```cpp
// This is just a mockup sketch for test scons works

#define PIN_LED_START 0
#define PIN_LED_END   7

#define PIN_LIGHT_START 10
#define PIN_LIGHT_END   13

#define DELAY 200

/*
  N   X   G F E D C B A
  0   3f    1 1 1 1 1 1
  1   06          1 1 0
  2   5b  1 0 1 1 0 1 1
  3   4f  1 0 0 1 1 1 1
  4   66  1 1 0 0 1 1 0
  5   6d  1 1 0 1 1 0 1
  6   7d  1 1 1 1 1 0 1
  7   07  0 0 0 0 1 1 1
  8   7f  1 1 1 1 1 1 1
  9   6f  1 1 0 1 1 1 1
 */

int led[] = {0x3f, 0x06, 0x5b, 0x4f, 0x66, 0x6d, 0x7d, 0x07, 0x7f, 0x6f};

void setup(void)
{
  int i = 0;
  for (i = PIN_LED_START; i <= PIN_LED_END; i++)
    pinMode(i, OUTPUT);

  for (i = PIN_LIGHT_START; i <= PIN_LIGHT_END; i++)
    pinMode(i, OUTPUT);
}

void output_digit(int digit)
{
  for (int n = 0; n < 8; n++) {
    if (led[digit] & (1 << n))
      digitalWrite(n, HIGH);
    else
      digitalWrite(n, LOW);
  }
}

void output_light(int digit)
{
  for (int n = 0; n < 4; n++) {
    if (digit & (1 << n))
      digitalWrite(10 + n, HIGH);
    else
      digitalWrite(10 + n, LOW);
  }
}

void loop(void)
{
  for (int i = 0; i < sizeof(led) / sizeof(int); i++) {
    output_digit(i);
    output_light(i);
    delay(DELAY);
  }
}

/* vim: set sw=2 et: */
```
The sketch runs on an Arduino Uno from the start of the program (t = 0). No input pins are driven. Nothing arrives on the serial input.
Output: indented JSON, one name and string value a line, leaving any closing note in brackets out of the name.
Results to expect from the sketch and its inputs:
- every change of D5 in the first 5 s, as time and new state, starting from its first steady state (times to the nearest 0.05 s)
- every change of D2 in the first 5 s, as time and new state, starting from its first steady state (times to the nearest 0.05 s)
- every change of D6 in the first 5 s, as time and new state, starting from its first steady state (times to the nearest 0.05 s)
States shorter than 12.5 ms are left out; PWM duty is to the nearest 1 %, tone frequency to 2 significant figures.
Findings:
{
  "every change of D5 in the first 5 s, as time and new state, starting from its first steady state": "0 s high; 0.2 s low; 0.8 s high; 1.4 s low; 1.6 s high; 2.2 s low; 2.8 s high; 3.4 s low; 3.6 s high; 4.2 s low; 4.8 s high",
  "every change of D2 in the first 5 s, as time and new state, starting from its first steady state": "0 s high; 0.4 s low; 0.6 s high; 2.4 s low; 2.6 s high; 4.4 s low; 4.6 s high",
  "every change of D6 in the first 5 s, as time and new state, starting from its first steady state": "0 s low; 0.4 s high; 1.4 s low; 1.6 s high; 2 s low; 2.4 s high; 3.4 s low; 3.6 s high; 4 s low; 4.4 s high"
}
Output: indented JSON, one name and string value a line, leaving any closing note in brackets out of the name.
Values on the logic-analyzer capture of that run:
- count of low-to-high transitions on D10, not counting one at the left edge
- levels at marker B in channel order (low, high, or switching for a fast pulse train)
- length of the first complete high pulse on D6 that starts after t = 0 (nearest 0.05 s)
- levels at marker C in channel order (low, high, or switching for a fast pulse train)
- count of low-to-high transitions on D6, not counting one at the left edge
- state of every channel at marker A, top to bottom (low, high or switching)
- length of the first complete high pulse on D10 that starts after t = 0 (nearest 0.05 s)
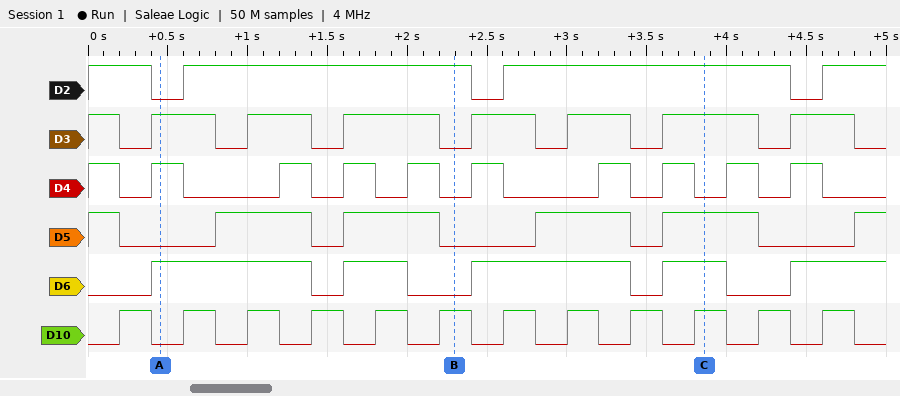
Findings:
{
  "count of low-to-high transitions on D10, not counting one at the left edge": "12",
  "levels at marker B in channel order": "D2 high, D3 low, D4 low, D5 low, D6 low, D10 high",
  "length of the first complete high pulse on D6 that starts after t = 0": "1.00 s",
  "levels at marker C in channel order": "D2 high, D3 high, D4 low, D5 high, D6 high, D10 high",
  "count of low-to-high transitions on D6, not counting one at the left edge": "5",
  "state of every channel at marker A, top to bottom": "D2 low, D3 high, D4 high, D5 low, D6 high, D10 low",
  "length of the first complete high pulse on D10 that starts after t = 0": "0.20 s"
}
